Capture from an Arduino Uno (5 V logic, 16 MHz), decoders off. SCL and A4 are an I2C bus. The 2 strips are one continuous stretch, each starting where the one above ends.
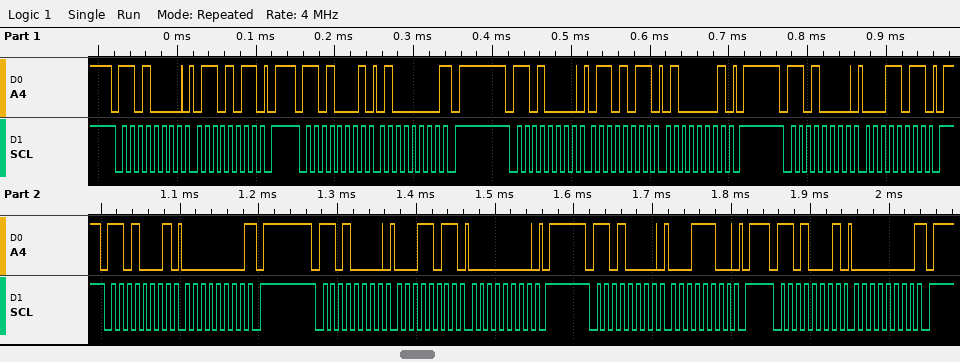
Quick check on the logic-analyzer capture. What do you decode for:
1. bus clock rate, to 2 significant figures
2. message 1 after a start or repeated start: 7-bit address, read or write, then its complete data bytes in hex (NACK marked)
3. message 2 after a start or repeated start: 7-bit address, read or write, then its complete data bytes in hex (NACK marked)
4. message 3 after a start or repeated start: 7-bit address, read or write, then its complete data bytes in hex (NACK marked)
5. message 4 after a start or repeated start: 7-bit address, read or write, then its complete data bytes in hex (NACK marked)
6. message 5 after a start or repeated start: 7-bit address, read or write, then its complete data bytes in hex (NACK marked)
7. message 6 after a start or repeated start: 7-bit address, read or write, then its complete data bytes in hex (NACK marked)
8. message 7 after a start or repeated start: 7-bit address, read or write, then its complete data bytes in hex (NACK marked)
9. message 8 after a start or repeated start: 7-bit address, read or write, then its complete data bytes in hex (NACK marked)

100 kHz
0x68 write: 6B
0x68 read: 40 NACK
0x68 write: 6B 41
0x68 write: 1B
0x68 read: 00 NACK
0x68 write: 1B 00
0x68 write: 1C
0x68 read: 00 NACK
